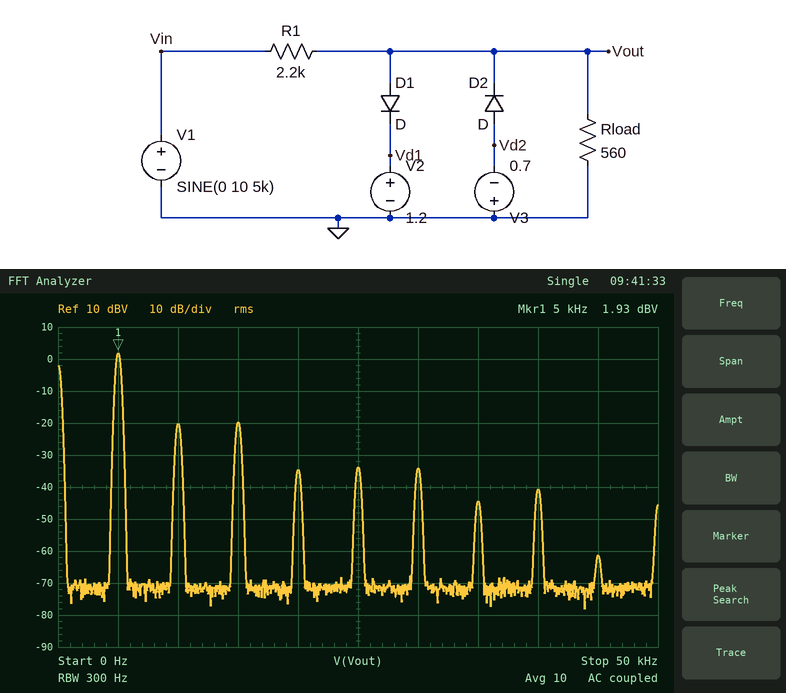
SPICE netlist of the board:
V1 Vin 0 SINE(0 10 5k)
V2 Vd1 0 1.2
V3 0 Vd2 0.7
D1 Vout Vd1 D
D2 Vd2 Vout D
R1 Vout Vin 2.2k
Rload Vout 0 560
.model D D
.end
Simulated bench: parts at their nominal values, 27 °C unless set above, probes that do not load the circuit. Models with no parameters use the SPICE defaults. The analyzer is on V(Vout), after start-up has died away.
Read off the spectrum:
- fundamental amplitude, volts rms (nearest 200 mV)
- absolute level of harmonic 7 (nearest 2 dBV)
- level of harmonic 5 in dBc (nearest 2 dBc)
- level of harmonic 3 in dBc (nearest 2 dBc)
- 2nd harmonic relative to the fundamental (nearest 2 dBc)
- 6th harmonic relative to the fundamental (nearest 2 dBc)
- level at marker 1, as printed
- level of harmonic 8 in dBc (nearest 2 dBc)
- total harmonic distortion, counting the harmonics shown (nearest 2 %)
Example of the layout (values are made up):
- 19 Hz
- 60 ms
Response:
- 1.2 V
- -44 dBV
- -36 dBc
- -22 dBc
- -22 dBc
- -36 dBc
- 1.93 dBV
- -42 dBc
- 12 %
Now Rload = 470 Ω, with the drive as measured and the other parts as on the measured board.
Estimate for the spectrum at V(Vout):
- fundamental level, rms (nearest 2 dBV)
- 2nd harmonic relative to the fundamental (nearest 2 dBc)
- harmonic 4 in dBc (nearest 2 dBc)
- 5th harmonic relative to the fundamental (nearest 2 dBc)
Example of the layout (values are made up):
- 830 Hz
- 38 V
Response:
- 2 dBV
- -24 dBc
- -32 dBc
- -38 dBc
